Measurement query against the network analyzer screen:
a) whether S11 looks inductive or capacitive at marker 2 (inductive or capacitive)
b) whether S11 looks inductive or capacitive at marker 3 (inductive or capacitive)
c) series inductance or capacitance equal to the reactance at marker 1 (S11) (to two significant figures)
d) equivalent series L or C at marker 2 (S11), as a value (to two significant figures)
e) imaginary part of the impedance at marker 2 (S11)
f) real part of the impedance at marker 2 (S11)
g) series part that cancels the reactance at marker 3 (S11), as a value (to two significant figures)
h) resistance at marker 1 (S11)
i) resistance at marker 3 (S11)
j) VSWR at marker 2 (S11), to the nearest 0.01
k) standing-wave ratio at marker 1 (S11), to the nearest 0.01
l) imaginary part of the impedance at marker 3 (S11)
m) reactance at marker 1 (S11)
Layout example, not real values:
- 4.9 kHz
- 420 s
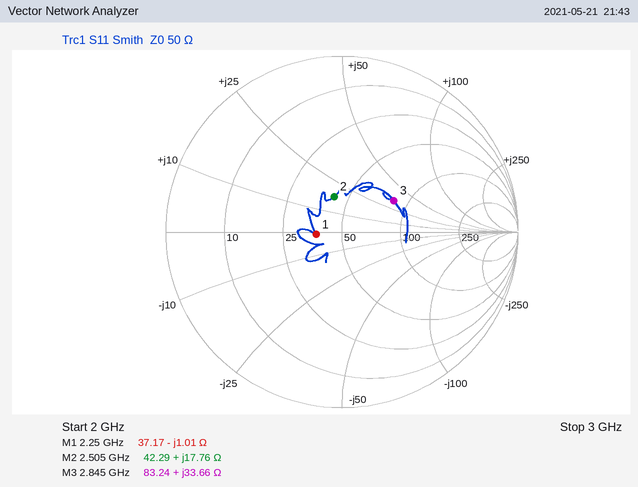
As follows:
- inductive
- inductive
- 70 pF
- 1.1 nH
- +17.76 Ω
- 42.29 Ω
- 1.7 pF
- 37.17 Ω
- 83.24 Ω
- 1.52
- 1.35
- +33.66 Ω
- -1.01 Ω
